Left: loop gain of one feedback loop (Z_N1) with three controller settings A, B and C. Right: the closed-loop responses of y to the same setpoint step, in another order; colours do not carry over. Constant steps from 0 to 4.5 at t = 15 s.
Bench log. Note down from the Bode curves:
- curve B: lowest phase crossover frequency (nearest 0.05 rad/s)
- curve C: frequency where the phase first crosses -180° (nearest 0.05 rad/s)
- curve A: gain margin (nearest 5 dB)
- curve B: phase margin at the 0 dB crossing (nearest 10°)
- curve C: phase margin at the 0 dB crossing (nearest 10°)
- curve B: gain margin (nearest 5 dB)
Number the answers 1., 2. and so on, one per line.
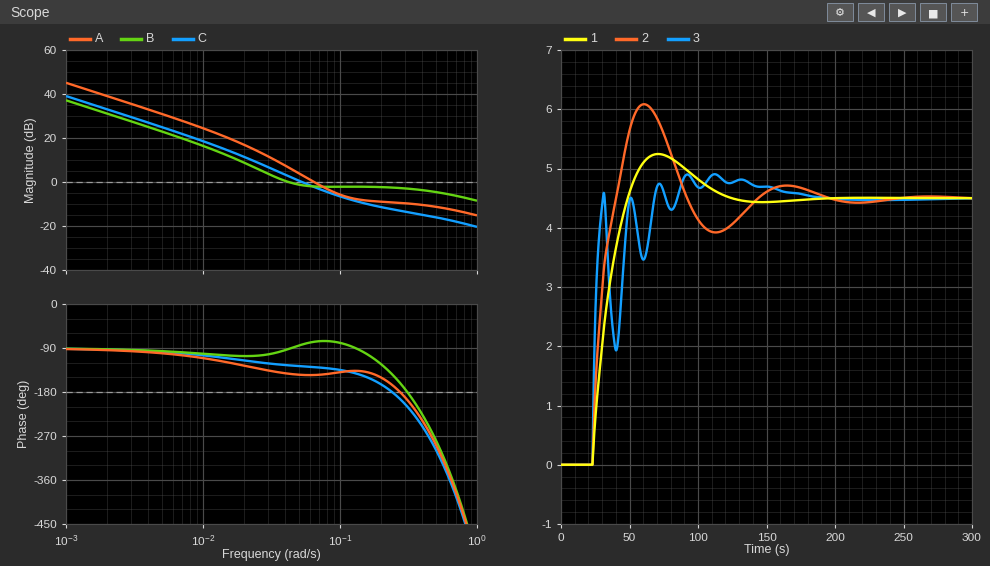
1. 0.30 rad/s
2. 0.25 rad/s
3. 10 dB
4. 90°
5. 50°
6. 5 dB
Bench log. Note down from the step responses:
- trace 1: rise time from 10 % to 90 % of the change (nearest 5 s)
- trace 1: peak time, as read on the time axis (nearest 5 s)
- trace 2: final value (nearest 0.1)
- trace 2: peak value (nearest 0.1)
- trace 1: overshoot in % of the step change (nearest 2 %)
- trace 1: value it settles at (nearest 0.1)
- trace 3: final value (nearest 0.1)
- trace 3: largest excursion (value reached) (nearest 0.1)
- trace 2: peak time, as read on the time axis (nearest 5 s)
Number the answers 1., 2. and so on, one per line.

1. 20 s
2. 70 s
3. 4.5
4. 6.1
5. 16 %
6. 4.5
7. 4.5
8. 4.9
9. 60 s
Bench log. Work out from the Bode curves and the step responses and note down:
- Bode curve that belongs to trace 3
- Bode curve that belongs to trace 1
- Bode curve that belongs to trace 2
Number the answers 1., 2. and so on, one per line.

1. B
2. C
3. A
